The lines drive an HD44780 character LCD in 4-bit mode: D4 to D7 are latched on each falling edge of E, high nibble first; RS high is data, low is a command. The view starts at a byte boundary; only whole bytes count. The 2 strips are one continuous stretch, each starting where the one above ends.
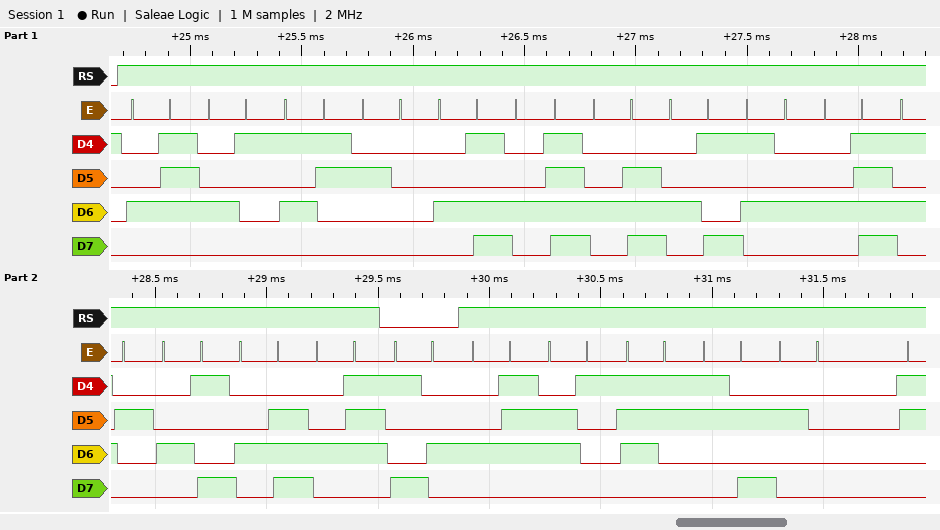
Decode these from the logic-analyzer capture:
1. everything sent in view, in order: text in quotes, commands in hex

"GAS MONITORING" 0x94 "Gas: "
